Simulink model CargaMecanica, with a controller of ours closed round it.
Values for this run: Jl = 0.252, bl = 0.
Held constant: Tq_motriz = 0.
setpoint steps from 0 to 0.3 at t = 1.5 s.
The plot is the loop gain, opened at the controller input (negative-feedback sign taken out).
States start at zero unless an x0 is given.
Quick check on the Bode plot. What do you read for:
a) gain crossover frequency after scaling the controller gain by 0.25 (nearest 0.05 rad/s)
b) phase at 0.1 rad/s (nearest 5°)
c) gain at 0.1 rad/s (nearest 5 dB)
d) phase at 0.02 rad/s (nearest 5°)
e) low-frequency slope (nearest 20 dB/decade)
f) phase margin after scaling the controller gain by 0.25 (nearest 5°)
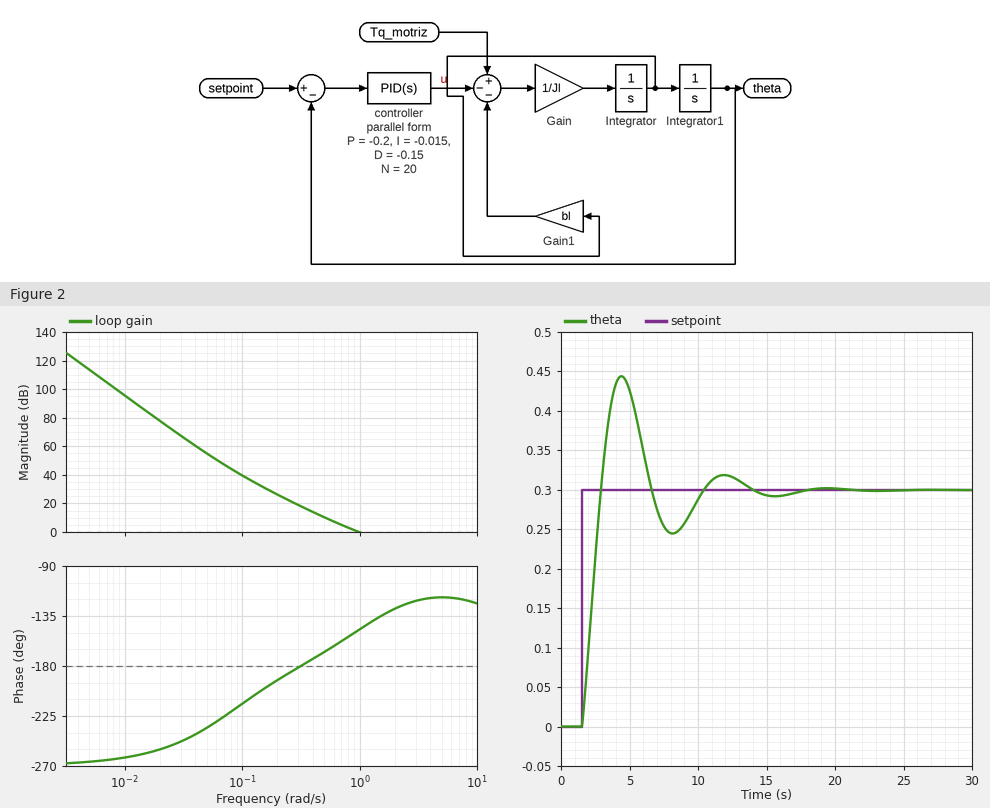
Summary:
0.45 rad/s
-215°
40 dB
-255°
-60 dB/decade
10°
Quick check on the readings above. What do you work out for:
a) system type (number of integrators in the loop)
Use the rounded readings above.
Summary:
3
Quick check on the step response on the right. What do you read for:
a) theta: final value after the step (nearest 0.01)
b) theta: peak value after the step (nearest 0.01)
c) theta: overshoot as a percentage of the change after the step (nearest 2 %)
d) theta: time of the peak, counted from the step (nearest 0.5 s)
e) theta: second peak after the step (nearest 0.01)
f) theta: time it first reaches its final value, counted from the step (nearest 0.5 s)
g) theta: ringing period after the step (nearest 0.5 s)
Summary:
0.30
0.44
48 %
3.0 s
0.32
1.5 s
7.5 s
